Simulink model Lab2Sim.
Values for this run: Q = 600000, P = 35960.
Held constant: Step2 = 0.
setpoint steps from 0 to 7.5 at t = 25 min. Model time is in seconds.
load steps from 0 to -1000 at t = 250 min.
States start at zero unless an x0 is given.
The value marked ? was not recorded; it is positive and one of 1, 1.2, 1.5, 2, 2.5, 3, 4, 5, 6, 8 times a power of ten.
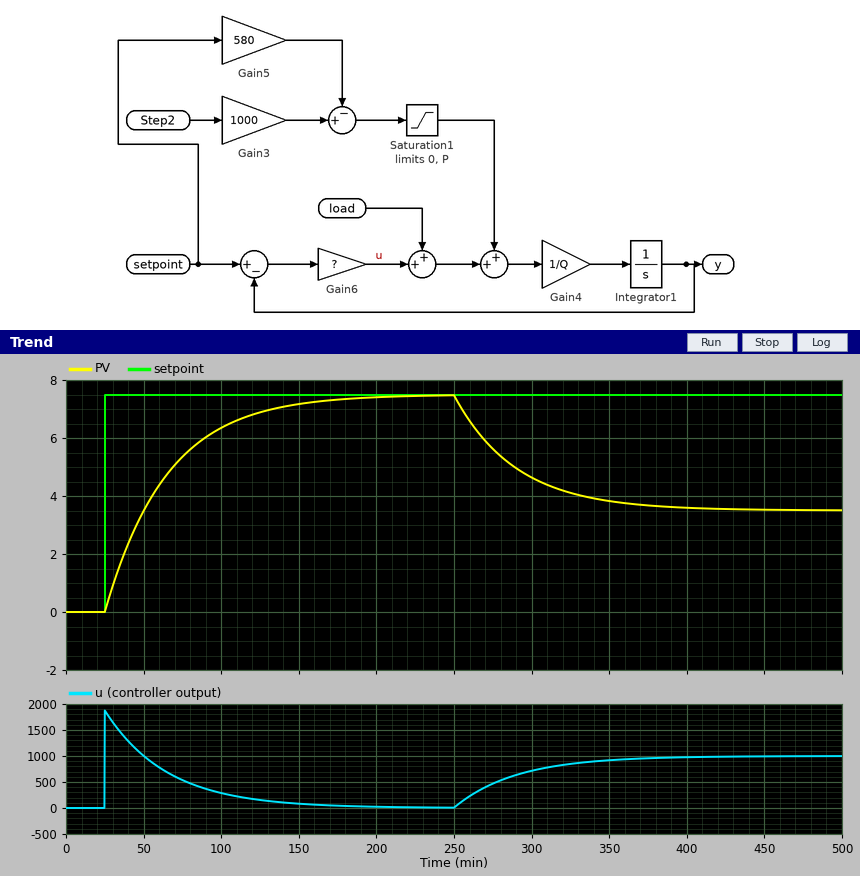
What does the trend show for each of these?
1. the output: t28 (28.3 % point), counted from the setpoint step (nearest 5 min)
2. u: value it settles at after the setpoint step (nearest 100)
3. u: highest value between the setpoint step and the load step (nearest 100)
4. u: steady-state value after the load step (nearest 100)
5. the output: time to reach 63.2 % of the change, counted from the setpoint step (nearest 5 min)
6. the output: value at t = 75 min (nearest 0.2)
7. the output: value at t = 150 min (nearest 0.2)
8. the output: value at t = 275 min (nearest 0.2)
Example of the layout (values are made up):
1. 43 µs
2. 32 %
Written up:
1. 15 min
2. 0
3. 1900
4. 1000
5. 40 min
6. 5.4
7. 7.2
8. 5.6
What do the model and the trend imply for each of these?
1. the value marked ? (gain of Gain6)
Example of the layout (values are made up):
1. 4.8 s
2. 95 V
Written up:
1. 250
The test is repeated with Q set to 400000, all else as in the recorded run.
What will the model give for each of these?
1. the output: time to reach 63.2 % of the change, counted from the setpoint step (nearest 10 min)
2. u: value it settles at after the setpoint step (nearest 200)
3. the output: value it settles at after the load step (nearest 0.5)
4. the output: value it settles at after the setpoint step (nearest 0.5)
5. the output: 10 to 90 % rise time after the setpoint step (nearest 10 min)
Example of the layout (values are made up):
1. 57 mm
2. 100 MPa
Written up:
1. 30 min
2. 0
3. 3.5
4. 7.5
5. 60 min
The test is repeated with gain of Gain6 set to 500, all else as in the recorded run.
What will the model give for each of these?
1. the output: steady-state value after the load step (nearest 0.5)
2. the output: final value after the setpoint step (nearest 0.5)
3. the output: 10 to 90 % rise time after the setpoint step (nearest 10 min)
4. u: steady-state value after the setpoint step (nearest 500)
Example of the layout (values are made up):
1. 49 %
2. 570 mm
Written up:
1. 5.5
2. 7.5
3. 40 min
4. 0
